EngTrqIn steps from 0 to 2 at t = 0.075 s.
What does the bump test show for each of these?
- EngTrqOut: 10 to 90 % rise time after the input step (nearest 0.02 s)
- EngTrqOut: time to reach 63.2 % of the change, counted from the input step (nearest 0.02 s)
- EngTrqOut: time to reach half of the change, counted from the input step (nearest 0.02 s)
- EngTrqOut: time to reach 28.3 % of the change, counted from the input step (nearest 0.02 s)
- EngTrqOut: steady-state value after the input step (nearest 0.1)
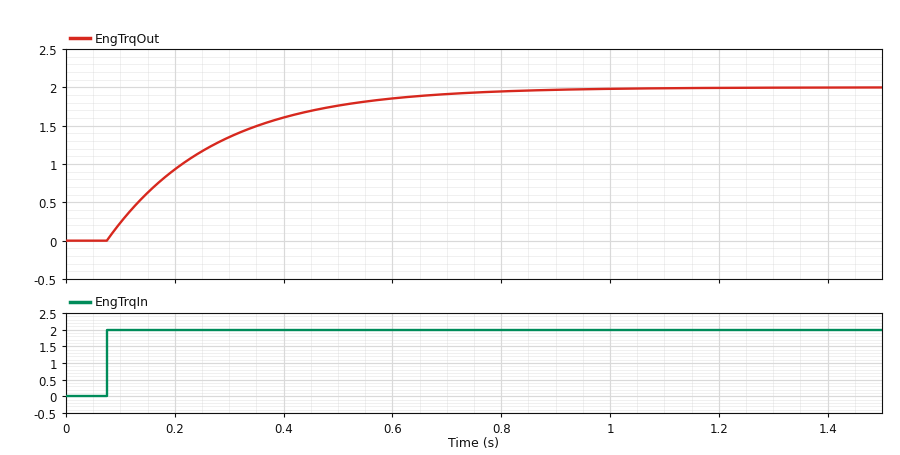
0.44 s
0.20 s
0.14 s
0.06 s
2.0
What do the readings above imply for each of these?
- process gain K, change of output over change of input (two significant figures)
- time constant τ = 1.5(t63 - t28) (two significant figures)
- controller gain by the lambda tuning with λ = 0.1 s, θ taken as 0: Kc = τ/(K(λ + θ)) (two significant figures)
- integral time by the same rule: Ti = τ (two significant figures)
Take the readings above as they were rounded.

1.0
0.21 s
2.1
0.21 s
